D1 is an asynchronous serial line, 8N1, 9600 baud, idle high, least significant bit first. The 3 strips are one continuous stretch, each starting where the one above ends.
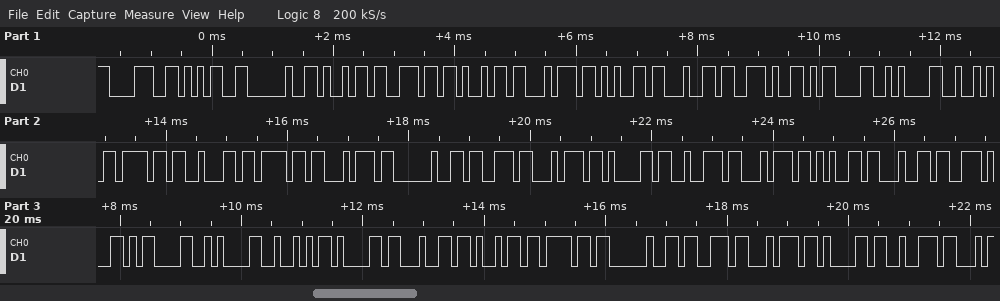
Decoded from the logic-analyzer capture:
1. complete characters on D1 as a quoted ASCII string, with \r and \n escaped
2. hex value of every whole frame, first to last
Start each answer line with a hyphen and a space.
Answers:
- "85 inited.\r\nRobot started.\r\nRadio star"
- 38 35 20 69 6E 69 74 65 64 2E 0D 0A 52 6F 62 6F 74 20 73 74 61 72 74 65 64 2E 0D 0A 52 61 64 69 6F 20 73 74 61 72
